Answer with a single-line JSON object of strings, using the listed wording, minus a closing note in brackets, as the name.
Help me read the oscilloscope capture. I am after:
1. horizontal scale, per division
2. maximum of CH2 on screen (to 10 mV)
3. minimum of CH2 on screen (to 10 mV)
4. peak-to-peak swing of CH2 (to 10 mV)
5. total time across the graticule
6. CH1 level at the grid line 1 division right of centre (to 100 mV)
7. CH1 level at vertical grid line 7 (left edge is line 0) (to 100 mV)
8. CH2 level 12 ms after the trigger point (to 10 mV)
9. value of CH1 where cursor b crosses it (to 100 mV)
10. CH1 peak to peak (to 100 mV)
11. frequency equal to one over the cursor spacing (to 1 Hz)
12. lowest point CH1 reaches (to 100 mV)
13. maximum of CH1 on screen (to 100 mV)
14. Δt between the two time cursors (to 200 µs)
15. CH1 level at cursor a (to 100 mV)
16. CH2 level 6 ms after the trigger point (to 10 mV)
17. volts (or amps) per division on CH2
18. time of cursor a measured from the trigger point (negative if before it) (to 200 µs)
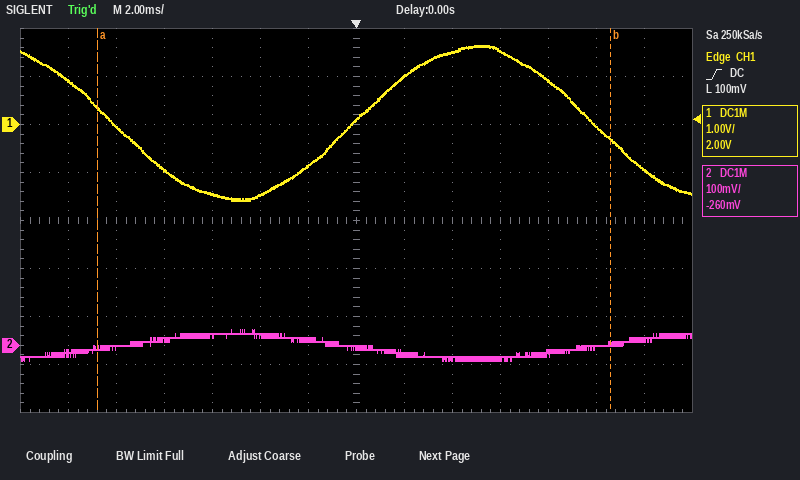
{"horizontal scale, per division": "2 ms", "maximum of CH2 on screen": "30 mV", "minimum of CH2 on screen": "-30 mV", "peak-to-peak swing of CH2": "60 mV", "total time across the graticule": "28 ms", "CH1 level at the grid line 1 division right of centre": "1.0 V", "CH1 level at vertical grid line 7 (left edge is line 0)": "100 mV", "CH2 level 12 ms after the trigger point": "10 mV", "value of CH1 where cursor b crosses it": "-300 mV", "CH1 peak to peak": "3.2 V", "frequency equal to one over the cursor spacing": "47 Hz", "lowest point CH1 reaches": "-1.6 V", "maximum of CH1 on screen": "1.6 V", "Δt between the two time cursors": "21.4 ms", "CH1 level at cursor a": "300 mV", "CH2 level 6 ms after the trigger point": "-30 mV", "volts (or amps) per division on CH2": "100 mV", "time of cursor a measured from the trigger point (negative if before it)": "-10.8 ms"}
